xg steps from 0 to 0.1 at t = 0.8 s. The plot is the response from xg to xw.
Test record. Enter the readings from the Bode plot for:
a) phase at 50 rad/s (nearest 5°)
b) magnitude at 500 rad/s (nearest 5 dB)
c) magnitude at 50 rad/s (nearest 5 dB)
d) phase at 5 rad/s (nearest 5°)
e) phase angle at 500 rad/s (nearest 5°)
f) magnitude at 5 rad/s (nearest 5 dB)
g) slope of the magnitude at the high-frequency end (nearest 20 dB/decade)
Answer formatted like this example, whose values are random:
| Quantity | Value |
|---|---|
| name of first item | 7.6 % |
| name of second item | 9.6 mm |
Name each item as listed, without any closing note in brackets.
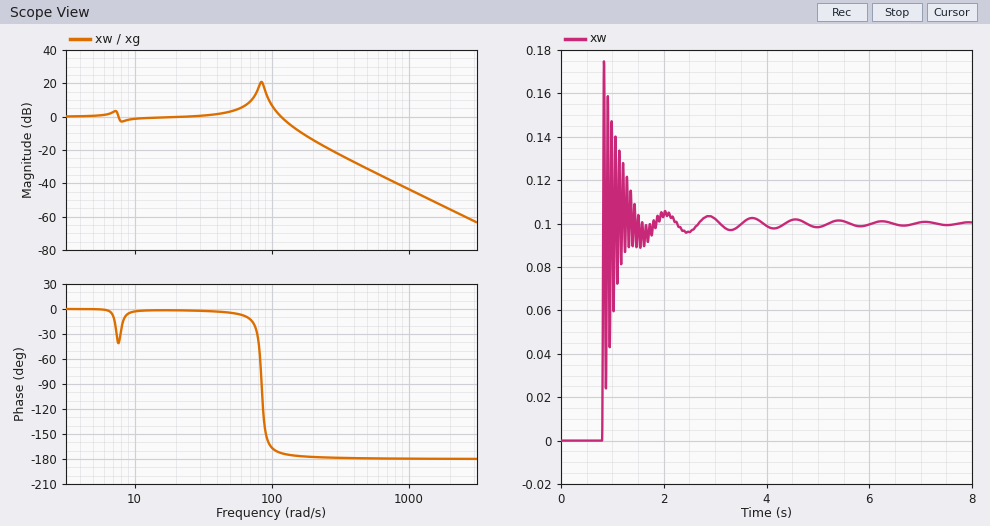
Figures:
| Quantity | Value |
|---|---|
| phase at 50 rad/s | -5° |
| magnitude at 500 rad/s | -30 dB |
| magnitude at 50 rad/s | 5 dB |
| phase at 5 rad/s | 0° |
| phase angle at 500 rad/s | -180° |
| magnitude at 5 rad/s | 0 dB |
| slope of the magnitude at the high-frequency end | -40 dB/decade |
